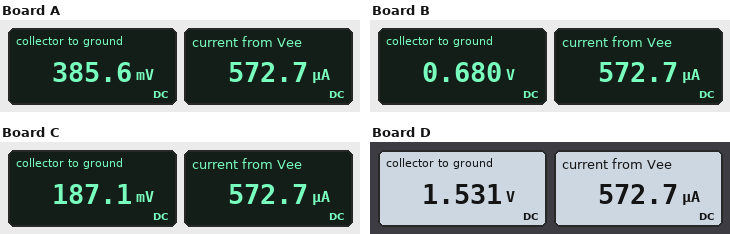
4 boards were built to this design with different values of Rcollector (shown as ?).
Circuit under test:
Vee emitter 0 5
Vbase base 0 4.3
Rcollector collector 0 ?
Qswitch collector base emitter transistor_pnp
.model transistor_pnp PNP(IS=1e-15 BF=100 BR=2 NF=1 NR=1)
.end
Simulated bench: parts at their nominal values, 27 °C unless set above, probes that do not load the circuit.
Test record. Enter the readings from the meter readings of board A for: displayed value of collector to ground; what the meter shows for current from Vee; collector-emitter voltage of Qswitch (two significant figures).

385.6 mV
572.7 µA
-4.6 V
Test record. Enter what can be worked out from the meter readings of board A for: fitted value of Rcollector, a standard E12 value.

680 Ω
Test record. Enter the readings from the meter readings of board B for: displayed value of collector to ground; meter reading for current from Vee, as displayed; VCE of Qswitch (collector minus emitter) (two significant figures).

0.680 V
572.7 µA
-4.3 V
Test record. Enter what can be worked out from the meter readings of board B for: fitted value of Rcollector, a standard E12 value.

1.2 kΩ
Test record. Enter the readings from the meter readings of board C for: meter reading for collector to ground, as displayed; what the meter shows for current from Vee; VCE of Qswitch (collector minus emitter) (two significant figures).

187.1 mV
572.7 µA
-4.8 V
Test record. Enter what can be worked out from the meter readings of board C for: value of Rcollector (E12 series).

330 Ω
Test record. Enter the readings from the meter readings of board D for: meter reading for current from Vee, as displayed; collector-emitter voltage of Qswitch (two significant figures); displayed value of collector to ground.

572.7 µA
-3.5 V
1.531 V
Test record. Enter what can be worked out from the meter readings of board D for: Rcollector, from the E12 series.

2.7 kΩ
